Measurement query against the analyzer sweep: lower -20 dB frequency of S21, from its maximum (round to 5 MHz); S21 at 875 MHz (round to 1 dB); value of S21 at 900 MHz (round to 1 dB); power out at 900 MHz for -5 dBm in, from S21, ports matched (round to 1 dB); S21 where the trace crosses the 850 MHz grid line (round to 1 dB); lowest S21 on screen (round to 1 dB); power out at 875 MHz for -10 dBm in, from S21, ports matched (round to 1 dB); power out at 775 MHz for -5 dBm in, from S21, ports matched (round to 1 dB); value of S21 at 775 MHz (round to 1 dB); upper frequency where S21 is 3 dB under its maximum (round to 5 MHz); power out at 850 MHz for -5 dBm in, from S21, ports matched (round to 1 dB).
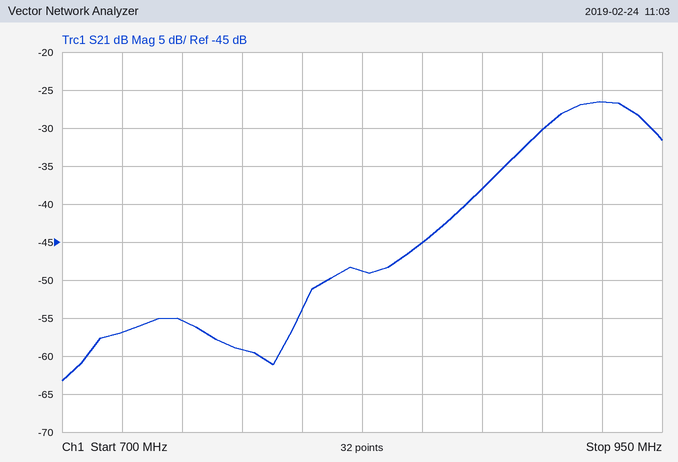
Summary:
845 MHz
-38 dB
-30 dB
-35 dBm
-45 dB
-63 dB
-48 dBm
-64 dBm
-59 dB
945 MHz
-50 dBm
